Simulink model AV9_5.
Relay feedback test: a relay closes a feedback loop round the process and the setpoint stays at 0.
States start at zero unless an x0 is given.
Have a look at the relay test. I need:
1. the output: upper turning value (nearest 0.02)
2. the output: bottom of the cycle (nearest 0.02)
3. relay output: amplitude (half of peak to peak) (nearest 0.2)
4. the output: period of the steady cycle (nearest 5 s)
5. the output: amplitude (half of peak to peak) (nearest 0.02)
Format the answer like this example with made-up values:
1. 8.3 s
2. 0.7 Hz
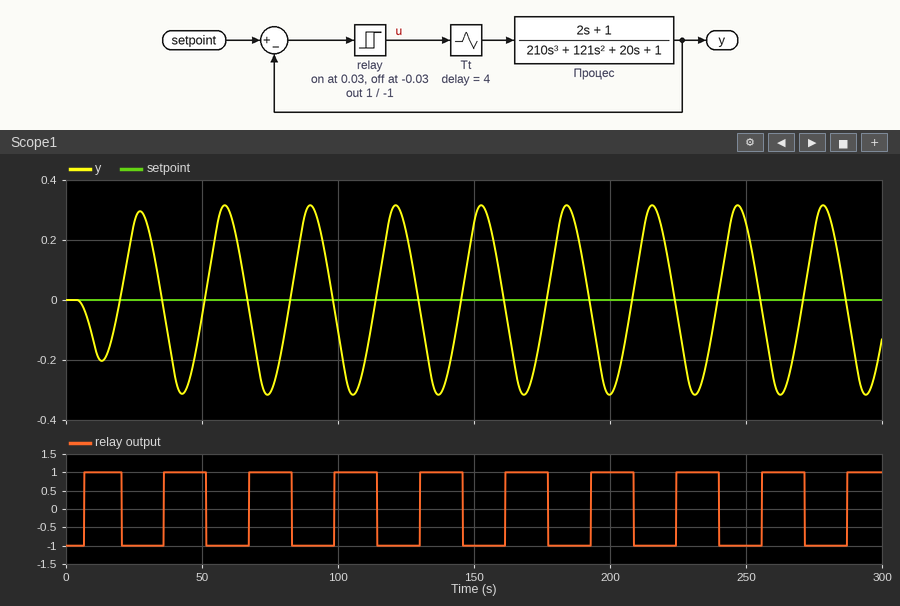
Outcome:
1. 0.32
2. -0.32
3. 1.0
4. 30 s
5. 0.32
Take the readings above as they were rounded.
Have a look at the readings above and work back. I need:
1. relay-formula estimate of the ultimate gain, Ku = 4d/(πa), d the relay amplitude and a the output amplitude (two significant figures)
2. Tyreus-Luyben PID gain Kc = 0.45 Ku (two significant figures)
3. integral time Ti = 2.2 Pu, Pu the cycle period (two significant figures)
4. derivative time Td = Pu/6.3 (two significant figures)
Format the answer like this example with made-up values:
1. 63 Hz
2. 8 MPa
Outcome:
1. 4.0
2. 1.8
3. 66 s
4. 4.8 s
